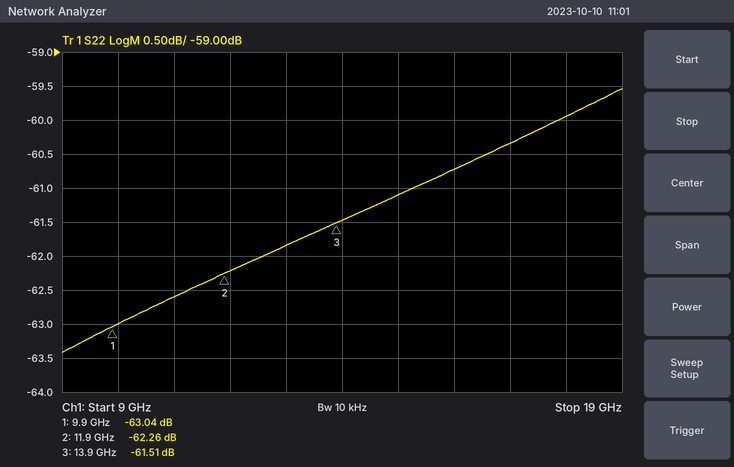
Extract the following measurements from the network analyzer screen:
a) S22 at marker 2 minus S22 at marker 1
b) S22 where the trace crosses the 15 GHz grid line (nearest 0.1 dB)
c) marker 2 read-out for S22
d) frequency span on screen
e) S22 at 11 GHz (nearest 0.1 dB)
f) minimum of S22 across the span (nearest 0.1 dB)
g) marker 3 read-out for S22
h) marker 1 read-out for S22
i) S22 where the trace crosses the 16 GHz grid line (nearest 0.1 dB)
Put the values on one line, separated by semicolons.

0.78 dB; -61.1 dB; -62.26 dB; 10 GHz; -62.6 dB; -63.4 dB; -61.51 dB; -63.04 dB; -60.7 dB
